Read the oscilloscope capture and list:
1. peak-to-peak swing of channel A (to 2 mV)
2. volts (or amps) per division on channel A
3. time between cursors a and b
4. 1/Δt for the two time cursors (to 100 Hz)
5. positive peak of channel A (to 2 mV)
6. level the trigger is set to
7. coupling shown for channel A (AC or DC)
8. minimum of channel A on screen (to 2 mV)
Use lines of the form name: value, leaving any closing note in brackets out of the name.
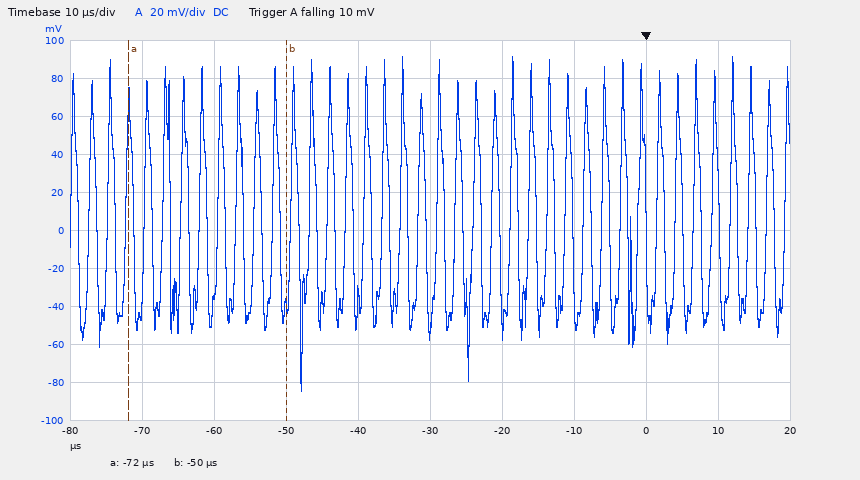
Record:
peak-to-peak swing of channel A: 176 mV
volts (or amps) per division on channel A: 20 mV
time between cursors a and b: 22 µs
1/Δt for the two time cursors: 45.5 kHz
positive peak of channel A: 92 mV
level the trigger is set to: 10 mV
coupling shown for channel A: DC
minimum of channel A on screen: -84 mV
